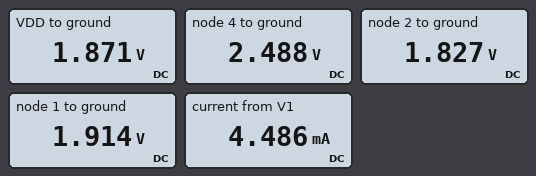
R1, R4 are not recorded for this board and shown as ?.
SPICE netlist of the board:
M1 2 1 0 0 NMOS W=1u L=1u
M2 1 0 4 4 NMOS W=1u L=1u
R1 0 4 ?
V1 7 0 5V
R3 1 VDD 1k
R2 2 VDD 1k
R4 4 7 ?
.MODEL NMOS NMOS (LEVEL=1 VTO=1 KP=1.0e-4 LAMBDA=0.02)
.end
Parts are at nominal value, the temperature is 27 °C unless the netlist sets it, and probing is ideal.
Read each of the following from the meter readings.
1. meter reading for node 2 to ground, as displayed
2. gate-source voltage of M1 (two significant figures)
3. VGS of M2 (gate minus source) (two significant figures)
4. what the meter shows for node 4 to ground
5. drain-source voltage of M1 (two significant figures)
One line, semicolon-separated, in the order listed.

1.827 V; 1.9 V; -2.5 V; 2.488 V; 1.8 V
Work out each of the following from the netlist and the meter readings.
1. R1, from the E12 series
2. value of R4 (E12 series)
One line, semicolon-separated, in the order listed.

560 Ω; 560 Ω
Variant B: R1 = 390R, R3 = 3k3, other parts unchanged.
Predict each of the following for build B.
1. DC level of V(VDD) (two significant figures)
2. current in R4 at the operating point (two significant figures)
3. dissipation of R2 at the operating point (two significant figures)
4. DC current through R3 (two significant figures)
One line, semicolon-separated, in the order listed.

1.5 V; 5.3 mA; 170 nW; 13 µA
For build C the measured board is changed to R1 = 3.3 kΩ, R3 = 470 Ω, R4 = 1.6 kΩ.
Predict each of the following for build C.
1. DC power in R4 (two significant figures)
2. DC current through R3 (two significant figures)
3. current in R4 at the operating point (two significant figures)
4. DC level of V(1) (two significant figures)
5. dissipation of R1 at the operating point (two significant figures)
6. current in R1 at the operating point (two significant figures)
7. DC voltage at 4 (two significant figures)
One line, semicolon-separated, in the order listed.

2.0 mW; 140 µA; 1.1 mA; 2.6 V; 3.1 mW; 980 µA; 3.2 V
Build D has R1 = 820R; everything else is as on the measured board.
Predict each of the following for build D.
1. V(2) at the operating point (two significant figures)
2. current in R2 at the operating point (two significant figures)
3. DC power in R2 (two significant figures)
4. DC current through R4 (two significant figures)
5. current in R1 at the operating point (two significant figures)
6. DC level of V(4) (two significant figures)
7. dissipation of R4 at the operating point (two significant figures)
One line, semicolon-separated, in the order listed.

2.2 V; 94 µA; 8.9 µW; 3.7 mA; 3.6 mA; 2.9 V; 7.6 mW
